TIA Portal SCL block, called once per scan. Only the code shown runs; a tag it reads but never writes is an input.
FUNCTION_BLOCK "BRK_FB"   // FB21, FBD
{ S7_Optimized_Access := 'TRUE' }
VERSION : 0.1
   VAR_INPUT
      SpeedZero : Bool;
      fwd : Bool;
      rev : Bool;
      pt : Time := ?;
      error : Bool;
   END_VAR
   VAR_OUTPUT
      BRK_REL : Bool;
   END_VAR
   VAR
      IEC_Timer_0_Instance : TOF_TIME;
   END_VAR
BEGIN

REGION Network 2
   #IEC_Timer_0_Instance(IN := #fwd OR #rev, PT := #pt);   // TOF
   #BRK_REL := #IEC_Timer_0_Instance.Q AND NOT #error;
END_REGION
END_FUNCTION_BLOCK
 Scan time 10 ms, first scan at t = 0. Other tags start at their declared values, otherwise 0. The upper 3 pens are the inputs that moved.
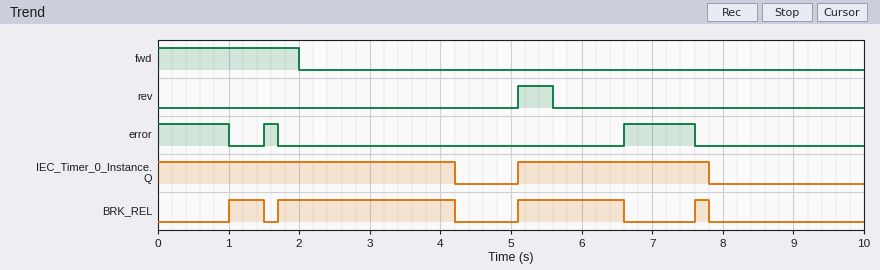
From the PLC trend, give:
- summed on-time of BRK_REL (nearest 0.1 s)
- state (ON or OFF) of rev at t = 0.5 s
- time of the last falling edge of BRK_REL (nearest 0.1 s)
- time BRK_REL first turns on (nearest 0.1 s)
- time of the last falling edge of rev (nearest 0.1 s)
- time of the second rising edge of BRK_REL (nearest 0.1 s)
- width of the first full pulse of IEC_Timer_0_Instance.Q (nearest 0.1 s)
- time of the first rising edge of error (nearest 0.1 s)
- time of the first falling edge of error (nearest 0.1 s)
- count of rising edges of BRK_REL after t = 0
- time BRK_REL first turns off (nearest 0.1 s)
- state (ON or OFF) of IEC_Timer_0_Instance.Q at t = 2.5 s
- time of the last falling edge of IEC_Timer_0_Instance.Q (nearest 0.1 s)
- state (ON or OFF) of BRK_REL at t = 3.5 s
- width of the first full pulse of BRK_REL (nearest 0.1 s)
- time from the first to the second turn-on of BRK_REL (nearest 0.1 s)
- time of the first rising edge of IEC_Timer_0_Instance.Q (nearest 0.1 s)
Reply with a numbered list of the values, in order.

1. 4.7 s
2. OFF
3. 7.8 s
4. 1.0 s
5. 5.6 s
6. 1.7 s
7. 2.7 s
8. 1.5 s
9. 1.0 s
10. 4
11. 1.5 s
12. ON
13. 7.8 s
14. ON
15. 0.5 s
16. 0.7 s
17. 5.1 s
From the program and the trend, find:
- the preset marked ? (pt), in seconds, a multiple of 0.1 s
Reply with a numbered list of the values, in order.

1. 2.2 s
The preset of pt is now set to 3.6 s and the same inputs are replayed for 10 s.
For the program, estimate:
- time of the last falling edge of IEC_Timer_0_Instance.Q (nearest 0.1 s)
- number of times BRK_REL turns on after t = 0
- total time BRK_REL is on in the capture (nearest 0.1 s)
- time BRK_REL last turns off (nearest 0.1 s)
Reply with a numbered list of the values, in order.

1. 9.2 s
2. 3
3. 7.0 s
4. 9.2 s
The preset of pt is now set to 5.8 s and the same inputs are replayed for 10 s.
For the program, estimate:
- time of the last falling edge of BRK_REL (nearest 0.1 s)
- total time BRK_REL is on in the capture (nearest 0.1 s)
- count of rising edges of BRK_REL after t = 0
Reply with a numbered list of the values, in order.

1. 6.6 s
2. 7.8 s
3. 3
